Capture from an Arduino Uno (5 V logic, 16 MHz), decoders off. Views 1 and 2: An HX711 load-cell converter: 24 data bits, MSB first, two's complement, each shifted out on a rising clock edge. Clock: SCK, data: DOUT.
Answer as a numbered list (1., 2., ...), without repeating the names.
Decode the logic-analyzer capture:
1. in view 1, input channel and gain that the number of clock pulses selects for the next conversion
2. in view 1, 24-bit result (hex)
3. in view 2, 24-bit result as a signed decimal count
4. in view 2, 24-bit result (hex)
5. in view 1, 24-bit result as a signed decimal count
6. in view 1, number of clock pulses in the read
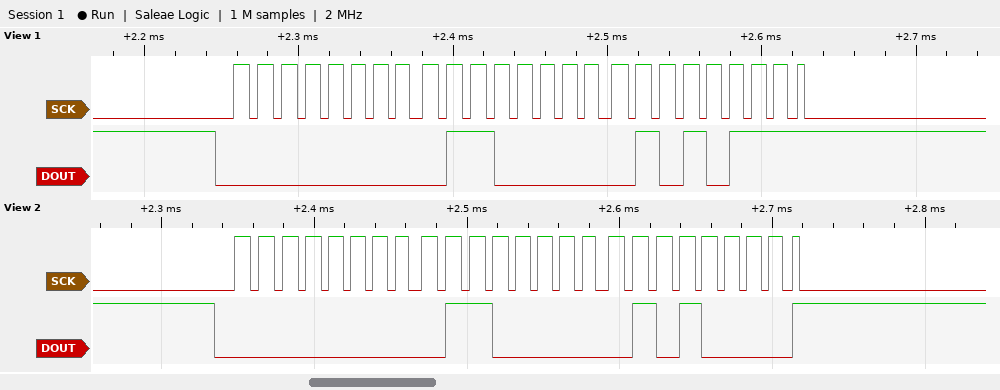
1. channel A, gain 128
2. 0x006057
3. 24656
4. 0x006050
5. 24663
6. 25
